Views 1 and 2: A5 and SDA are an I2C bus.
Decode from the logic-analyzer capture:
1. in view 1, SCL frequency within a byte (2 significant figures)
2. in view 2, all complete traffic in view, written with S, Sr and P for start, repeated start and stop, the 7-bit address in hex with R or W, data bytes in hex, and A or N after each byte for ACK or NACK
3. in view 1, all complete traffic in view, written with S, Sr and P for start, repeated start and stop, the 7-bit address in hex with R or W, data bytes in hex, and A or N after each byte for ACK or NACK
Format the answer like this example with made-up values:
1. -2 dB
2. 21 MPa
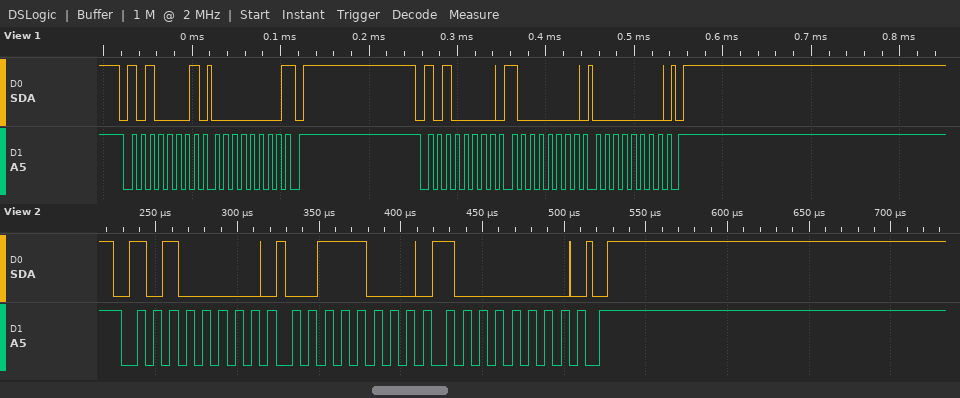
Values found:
1. 100 kHz
2. S 50W A 38 A 80 A P
3. S 50R A 00 N P S 50W A 80 A 00 A P
